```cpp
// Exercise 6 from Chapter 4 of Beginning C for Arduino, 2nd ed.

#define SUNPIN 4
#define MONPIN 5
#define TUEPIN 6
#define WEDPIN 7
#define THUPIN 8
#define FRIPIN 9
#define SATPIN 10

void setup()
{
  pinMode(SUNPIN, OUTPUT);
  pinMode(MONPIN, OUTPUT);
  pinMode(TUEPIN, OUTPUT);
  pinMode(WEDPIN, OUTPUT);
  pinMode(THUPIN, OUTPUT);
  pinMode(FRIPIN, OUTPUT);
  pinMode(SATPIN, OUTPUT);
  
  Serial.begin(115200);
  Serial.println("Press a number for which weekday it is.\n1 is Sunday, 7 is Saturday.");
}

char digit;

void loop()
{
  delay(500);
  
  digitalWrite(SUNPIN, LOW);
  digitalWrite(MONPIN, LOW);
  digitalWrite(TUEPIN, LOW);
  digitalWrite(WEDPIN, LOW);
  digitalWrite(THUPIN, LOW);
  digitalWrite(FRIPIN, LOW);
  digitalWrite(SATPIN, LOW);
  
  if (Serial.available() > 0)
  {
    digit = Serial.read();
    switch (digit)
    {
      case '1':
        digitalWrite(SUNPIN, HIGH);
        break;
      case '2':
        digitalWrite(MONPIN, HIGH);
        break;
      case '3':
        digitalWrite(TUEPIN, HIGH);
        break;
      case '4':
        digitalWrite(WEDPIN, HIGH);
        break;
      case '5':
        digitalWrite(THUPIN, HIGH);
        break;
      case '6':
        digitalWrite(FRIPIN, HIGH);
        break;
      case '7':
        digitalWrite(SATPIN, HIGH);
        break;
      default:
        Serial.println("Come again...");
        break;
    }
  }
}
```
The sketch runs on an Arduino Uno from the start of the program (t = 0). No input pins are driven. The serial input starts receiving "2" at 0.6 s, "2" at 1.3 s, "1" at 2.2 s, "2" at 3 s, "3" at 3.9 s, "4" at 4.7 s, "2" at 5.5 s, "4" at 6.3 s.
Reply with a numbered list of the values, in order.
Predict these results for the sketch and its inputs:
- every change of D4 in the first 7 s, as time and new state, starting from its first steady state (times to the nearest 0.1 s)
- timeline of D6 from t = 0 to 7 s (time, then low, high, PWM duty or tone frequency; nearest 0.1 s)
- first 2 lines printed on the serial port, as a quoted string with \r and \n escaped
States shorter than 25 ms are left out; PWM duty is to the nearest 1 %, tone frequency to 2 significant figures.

1. 0 s low; 2.5 s high; 3 s low
2. 0 s low; 4 s high; 4.5 s low
3. "Press a number for which weekday it is.\n1 is Sunday, 7 is Saturday.\r\n"
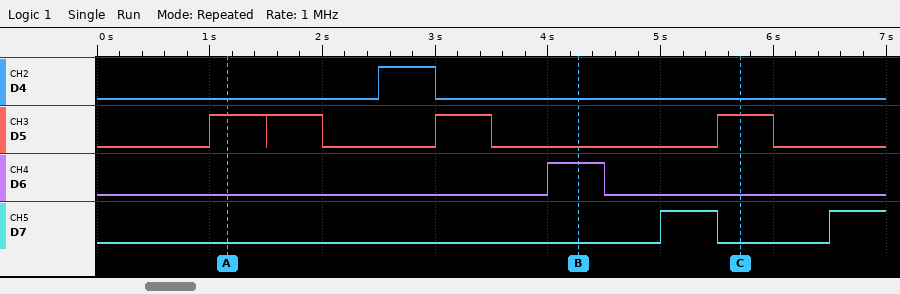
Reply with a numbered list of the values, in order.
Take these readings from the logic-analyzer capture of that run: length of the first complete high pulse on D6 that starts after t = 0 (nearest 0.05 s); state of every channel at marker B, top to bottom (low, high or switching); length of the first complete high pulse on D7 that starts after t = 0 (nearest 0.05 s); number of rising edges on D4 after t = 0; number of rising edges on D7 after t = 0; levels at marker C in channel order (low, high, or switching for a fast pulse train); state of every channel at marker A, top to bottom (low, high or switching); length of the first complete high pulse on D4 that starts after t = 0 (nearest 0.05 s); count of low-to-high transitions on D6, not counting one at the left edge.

1. 0.50 s
2. D4 low, D5 low, D6 high, D7 low
3. 0.50 s
4. 1
5. 2
6. D4 low, D5 high, D6 low, D7 low
7. D4 low, D5 high, D6 low, D7 low
8. 0.50 s
9. 1
